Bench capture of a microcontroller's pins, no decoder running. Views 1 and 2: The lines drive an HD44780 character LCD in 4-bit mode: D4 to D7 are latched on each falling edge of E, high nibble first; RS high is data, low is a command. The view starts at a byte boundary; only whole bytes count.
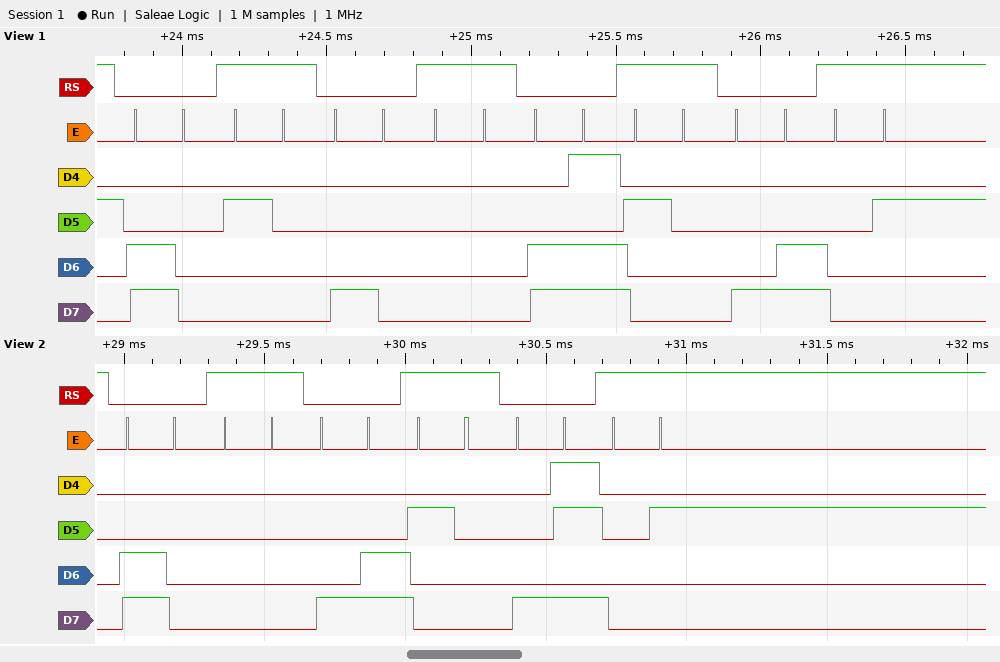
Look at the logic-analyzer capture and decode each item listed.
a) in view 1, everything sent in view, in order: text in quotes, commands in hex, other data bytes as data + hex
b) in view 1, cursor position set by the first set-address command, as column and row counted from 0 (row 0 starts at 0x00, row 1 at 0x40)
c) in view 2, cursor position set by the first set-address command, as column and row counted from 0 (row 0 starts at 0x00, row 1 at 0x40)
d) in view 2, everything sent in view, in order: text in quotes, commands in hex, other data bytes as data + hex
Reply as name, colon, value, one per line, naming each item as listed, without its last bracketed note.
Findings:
in view 1, everything sent in view, in order: text in quotes, commands in hex, other data bytes as data + hex: 0xC0 " " 0x80 data 00 0xCD " " 0x8C data 02
in view 1, cursor position set by the first set-address command, as column and row counted from 0: column 0, row 1
in view 2, cursor position set by the first set-address command, as column and row counted from 0: column 0, row 1
in view 2, everything sent in view, in order: text in quotes, commands in hex, other data bytes as data + hex: 0xC0 data 00 0x8C " " 0x8B data 02
